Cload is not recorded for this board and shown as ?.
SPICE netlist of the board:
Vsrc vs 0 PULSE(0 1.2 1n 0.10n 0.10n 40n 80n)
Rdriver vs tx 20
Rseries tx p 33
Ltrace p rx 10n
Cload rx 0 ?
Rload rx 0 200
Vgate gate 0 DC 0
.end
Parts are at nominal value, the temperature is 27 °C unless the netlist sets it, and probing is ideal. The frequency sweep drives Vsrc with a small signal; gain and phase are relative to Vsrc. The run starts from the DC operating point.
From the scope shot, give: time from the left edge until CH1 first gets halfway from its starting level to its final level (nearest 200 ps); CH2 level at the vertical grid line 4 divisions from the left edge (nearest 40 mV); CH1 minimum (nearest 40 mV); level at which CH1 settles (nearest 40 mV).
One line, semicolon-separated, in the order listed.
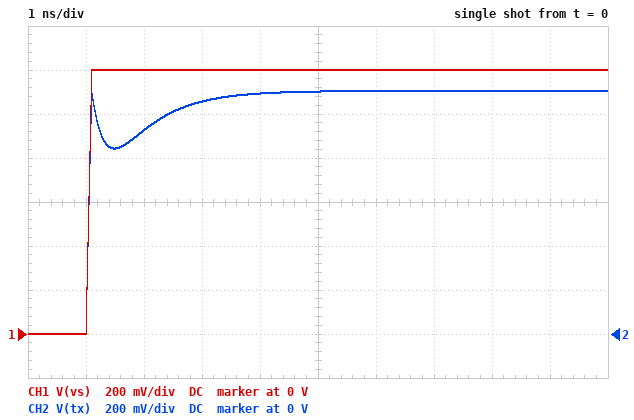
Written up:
1.0 ns; 1.08 V; 0 V; 1.20 V
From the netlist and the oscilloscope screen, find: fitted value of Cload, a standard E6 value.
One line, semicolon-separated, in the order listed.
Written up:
22 pF
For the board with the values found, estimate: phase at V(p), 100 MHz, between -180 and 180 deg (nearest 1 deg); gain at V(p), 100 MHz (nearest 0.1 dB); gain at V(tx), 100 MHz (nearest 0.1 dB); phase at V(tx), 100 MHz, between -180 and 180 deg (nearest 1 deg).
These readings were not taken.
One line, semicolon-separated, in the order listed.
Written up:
-31 deg; -3.7 dB; -1.5 dB; -9 deg
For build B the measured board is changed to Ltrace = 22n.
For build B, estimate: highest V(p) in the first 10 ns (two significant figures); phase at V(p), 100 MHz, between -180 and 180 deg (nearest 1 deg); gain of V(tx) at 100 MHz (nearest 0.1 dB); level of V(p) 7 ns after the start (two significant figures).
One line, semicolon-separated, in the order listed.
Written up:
1.1 V; -32 deg; -1.7 dB; 950 mV
